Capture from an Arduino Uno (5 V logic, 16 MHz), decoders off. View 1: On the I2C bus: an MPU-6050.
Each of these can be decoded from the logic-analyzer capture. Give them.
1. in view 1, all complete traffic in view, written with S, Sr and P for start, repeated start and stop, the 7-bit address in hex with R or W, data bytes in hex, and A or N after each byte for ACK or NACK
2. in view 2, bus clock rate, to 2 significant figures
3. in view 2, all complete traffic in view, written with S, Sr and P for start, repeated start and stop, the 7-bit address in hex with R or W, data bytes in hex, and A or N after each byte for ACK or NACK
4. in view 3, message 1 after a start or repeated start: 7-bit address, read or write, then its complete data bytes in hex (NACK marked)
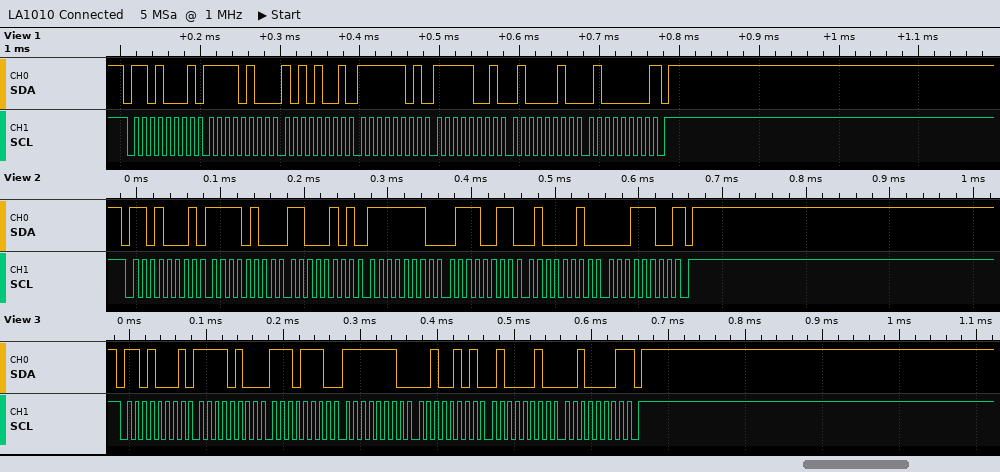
S 68R A F4 A A9 A FD A F9 A 42 A 40 N P
100 kHz
S 68R A F4 A C5 A FE A 73 A 42 A 1C N P
0x68 read: F4 EE FE 25 42 21 NACK
